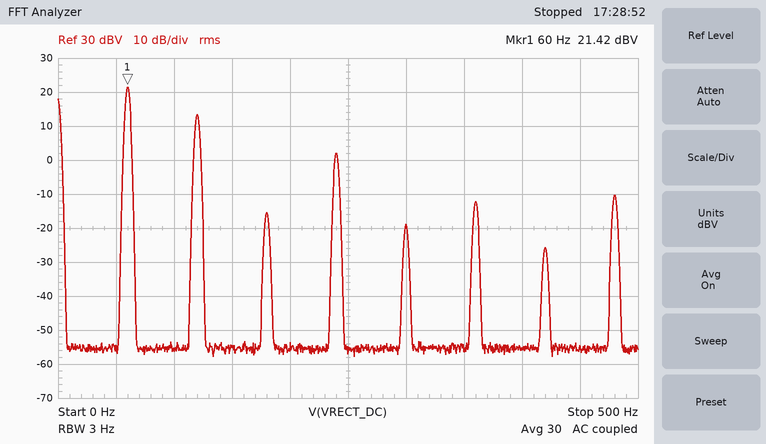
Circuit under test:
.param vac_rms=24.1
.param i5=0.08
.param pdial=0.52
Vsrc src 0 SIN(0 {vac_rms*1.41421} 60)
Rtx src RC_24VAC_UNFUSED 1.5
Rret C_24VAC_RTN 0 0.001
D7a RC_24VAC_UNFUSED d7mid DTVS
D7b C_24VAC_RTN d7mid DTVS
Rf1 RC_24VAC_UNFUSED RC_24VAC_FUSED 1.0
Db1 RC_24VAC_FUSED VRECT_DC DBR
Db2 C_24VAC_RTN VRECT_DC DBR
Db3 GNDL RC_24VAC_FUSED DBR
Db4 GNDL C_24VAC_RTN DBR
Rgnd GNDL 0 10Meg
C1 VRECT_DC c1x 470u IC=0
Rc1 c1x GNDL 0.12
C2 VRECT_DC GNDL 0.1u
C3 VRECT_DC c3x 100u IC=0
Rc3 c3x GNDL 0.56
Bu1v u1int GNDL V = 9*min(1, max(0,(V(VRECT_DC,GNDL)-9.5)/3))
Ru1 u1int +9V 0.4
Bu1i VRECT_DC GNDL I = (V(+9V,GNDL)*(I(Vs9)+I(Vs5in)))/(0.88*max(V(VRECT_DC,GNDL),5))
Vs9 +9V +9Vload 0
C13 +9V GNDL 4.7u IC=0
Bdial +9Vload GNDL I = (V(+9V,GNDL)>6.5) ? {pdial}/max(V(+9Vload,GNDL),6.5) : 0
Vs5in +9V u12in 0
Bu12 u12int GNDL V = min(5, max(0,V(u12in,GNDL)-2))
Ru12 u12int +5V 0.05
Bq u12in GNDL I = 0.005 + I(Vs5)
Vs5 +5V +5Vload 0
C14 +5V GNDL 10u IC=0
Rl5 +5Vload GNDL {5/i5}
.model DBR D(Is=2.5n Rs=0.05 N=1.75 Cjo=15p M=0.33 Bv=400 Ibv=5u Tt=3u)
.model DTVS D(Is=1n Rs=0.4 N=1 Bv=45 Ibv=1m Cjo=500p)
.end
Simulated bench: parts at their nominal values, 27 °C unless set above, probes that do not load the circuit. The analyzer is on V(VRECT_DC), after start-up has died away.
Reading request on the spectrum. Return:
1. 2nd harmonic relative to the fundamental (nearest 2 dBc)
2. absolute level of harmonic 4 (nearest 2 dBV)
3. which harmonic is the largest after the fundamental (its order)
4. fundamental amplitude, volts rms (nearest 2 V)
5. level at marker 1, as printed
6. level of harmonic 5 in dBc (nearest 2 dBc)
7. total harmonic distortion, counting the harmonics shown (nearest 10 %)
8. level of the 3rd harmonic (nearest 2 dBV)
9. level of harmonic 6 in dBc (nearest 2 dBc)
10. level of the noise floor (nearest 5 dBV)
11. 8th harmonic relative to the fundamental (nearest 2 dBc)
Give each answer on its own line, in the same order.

-8 dBc
2 dBV
2
12 V
21.42 dBV
-40 dBc
40 %
-16 dBV
-34 dBc
-55 dBV
-32 dBc
